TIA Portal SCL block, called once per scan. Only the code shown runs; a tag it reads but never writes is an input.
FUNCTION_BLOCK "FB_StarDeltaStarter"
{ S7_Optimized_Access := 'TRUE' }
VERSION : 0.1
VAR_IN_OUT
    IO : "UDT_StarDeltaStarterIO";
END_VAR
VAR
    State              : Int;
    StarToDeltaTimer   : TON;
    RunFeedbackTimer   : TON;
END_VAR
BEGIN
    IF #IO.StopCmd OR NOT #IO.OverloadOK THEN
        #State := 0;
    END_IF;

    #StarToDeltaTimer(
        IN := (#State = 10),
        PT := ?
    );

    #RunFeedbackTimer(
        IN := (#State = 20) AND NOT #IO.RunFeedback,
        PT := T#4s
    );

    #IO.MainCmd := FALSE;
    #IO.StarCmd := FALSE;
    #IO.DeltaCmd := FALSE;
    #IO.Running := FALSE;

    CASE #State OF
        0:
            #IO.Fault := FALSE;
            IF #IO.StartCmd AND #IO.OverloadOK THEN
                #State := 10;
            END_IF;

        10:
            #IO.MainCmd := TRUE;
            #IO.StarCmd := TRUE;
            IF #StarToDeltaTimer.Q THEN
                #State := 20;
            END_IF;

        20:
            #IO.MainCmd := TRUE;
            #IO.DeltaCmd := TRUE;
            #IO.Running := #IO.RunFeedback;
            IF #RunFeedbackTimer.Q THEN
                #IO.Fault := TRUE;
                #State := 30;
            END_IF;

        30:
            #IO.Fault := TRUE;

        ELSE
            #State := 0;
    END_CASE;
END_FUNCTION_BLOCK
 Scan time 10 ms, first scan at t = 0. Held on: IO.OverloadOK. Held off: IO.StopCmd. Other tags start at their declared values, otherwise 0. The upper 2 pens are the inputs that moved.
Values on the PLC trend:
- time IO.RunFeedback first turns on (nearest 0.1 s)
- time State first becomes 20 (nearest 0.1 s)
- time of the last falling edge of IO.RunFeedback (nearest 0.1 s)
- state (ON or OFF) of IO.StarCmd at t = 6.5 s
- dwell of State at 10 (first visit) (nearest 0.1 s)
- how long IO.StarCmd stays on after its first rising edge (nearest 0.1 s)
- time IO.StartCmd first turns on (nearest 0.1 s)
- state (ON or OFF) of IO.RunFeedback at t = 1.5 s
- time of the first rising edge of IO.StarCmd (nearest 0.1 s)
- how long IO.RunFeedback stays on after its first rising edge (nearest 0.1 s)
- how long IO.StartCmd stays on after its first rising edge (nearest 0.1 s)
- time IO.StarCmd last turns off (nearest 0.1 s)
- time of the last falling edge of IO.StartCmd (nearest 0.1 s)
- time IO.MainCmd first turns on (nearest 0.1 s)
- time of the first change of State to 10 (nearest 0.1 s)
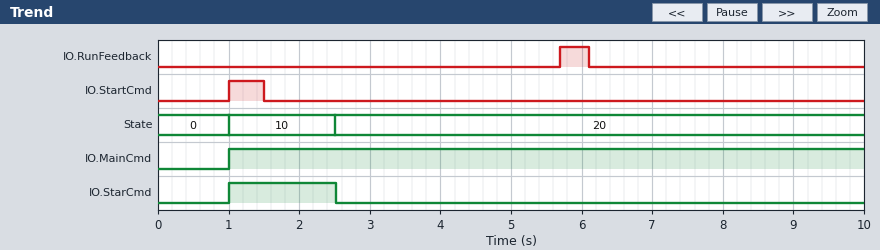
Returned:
5.7 s
2.5 s
6.1 s
OFF
1.5 s
1.5 s
1.0 s
OFF
1.0 s
0.4 s
0.5 s
2.5 s
1.5 s
1.0 s
1.0 s
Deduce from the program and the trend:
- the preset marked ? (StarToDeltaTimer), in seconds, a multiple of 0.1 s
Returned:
1.5 s
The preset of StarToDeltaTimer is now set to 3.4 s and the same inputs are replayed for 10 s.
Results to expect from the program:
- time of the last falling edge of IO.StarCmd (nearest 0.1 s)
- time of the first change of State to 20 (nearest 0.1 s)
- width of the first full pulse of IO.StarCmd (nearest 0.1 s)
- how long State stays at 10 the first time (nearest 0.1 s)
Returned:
4.4 s
4.4 s
3.4 s
3.4 s
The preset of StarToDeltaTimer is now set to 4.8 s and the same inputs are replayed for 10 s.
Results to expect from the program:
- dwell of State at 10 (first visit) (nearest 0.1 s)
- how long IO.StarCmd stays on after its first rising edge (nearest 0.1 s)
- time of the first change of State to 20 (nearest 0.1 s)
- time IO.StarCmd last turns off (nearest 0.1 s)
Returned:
4.8 s
4.8 s
5.8 s
5.8 s
